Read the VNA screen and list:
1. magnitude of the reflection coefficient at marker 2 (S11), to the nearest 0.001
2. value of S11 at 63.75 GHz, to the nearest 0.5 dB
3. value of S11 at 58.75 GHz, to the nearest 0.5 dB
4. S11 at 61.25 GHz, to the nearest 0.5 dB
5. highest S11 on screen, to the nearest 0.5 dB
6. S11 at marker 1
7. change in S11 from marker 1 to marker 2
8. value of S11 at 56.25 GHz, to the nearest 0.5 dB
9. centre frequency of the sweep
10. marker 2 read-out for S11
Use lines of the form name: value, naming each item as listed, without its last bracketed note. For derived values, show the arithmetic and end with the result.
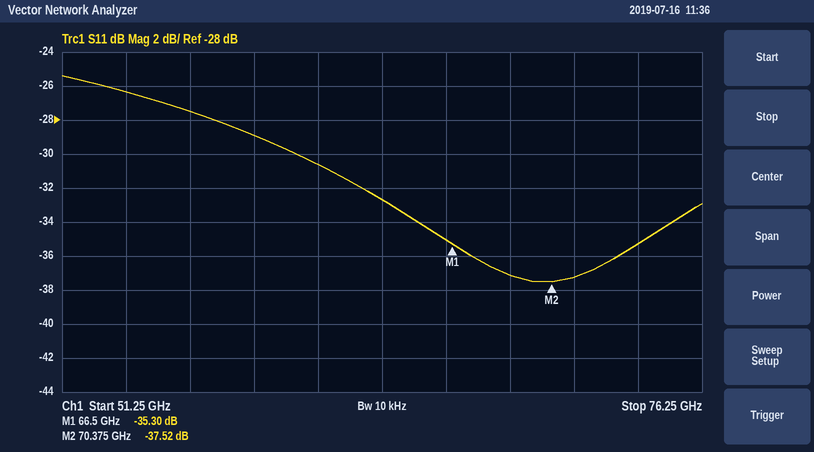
magnitude of the reflection coefficient at marker 2 (S11), to the nearest 0.001: 10^(-37.52/20) ≈ 0.013
value of S11 at 63.75 GHz, to the nearest 0.5 dB: -32.5 dB
value of S11 at 58.75 GHz, to the nearest 0.5 dB: -29.0 dB
S11 at 61.25 GHz, to the nearest 0.5 dB: -30.5 dB
highest S11 on screen, to the nearest 0.5 dB: -25.5 dB
S11 at marker 1: -35.30 dB
change in S11 from marker 1 to marker 2: -37.52 − (-35.3) = -2.22 dB
value of S11 at 56.25 GHz, to the nearest 0.5 dB: -27.5 dB
centre frequency of the sweep: 63.75 GHz
marker 2 read-out for S11: -37.52 dB
